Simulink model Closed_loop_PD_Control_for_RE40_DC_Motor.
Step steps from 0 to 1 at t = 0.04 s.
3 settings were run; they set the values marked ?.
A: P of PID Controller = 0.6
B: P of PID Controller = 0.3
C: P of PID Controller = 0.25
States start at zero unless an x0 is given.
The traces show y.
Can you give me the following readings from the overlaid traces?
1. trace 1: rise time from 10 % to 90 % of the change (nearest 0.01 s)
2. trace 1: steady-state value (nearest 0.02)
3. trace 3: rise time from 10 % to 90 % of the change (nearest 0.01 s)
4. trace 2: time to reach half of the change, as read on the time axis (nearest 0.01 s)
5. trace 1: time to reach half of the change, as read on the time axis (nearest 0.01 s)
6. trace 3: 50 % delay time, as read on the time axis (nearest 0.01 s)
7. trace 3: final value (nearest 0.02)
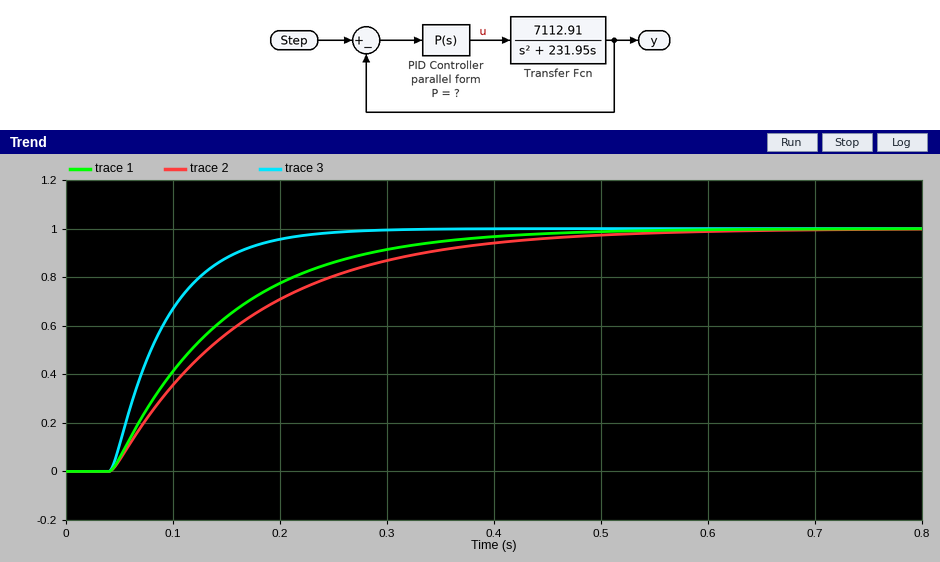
0.23 s
1.00
0.11 s
0.13 s
0.12 s
0.08 s
1.00
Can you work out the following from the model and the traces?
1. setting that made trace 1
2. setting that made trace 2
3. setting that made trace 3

B
C
A
